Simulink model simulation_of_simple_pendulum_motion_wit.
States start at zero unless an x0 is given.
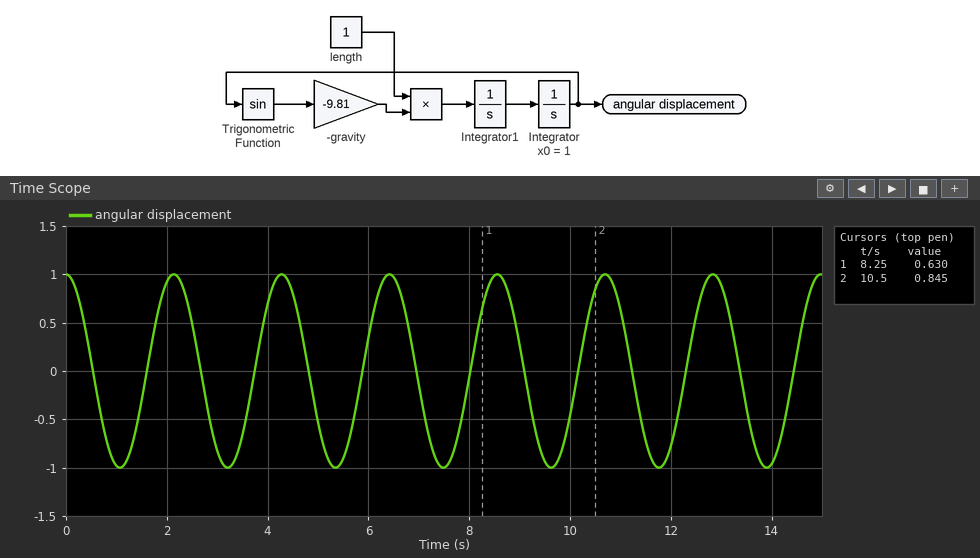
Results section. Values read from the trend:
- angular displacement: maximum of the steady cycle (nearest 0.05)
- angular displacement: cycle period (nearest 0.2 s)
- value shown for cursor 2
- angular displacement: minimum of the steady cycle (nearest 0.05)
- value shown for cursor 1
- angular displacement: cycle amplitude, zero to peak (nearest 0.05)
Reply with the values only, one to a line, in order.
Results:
1.00
2.2 s
0.845
-1.00
0.630
1.00
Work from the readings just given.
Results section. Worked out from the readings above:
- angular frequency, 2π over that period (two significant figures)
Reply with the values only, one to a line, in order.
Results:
2.9 rad/s
